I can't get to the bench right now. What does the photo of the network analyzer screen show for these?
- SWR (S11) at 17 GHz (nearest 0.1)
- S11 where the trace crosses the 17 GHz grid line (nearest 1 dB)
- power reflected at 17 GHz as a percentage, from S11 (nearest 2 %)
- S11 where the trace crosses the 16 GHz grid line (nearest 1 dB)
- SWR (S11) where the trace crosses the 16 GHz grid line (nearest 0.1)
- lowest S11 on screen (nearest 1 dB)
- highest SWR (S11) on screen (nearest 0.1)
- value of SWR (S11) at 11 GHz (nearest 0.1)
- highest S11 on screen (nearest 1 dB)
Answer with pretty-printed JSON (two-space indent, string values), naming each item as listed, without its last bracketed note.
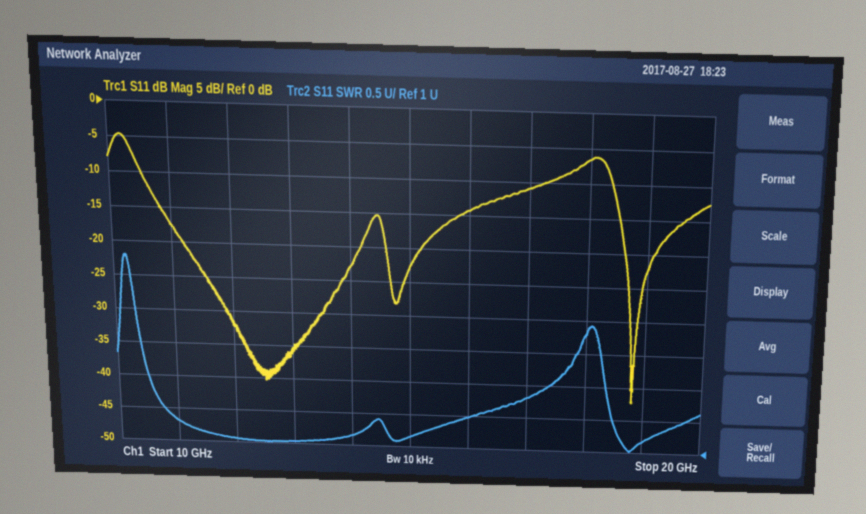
{
  "SWR (S11) at 17 GHz": "1.8",
  "S11 where the trace crosses the 17 GHz grid line": "-11 dB",
  "power reflected at 17 GHz as a percentage, from S11": "8 %",
  "S11 where the trace crosses the 16 GHz grid line": "-14 dB",
  "SWR (S11) where the trace crosses the 16 GHz grid line": "1.5",
  "lowest S11 on screen": "-42 dB",
  "highest SWR (S11) on screen": "3.8",
  "value of SWR (S11) at 11 GHz": "1.3",
  "highest S11 on screen": "-5 dB"
}
